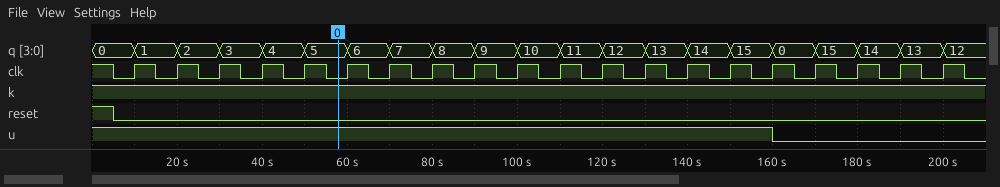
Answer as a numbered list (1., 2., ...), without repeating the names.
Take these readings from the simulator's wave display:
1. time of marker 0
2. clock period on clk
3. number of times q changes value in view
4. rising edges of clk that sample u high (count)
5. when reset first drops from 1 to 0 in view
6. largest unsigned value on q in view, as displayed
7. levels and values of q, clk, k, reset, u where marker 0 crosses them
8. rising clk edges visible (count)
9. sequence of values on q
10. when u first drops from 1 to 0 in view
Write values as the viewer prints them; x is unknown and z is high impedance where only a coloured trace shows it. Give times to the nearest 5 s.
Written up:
1. 60 s
2. 10 s
3. 20
4. 16
5. 5 s
6. 15
7. q=5, clk=0, k=1, reset=0, u=1
8. 20
9. 0, 1, 2, 3, 4, 5, 6, 7, 8, 9, 10, 11, 12, 13, 14, 15, 0, 15, 14, 13, 12
10. 160 s
